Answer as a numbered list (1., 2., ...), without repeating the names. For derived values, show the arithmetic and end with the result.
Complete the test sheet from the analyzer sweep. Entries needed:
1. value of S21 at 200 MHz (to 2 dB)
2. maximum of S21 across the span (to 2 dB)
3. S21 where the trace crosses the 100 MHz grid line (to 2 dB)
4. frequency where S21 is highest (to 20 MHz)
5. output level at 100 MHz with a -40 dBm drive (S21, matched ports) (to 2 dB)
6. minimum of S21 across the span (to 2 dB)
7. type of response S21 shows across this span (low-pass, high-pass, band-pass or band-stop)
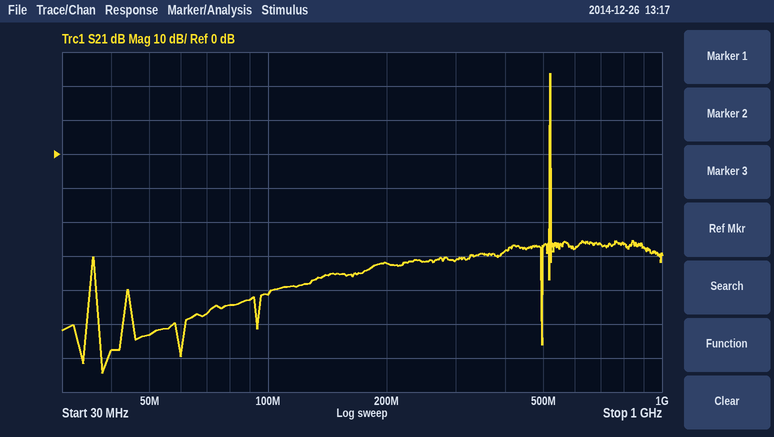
1. -32 dB
2. 24 dB
3. -42 dB
4. 520 MHz
5. -40 dBm + (-42 dB) = -82 dBm
6. -64 dB
7. band-pass
